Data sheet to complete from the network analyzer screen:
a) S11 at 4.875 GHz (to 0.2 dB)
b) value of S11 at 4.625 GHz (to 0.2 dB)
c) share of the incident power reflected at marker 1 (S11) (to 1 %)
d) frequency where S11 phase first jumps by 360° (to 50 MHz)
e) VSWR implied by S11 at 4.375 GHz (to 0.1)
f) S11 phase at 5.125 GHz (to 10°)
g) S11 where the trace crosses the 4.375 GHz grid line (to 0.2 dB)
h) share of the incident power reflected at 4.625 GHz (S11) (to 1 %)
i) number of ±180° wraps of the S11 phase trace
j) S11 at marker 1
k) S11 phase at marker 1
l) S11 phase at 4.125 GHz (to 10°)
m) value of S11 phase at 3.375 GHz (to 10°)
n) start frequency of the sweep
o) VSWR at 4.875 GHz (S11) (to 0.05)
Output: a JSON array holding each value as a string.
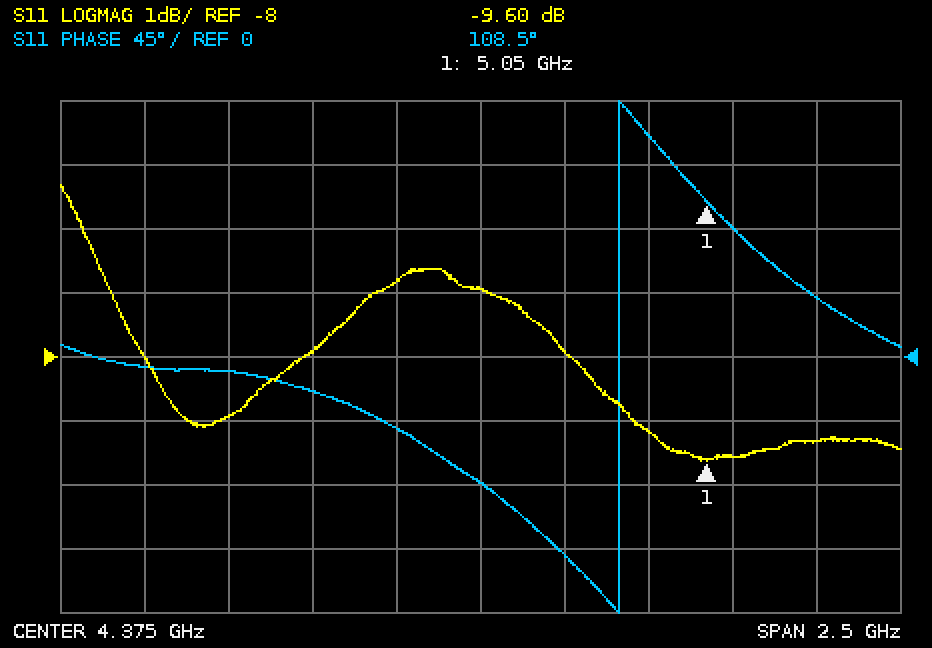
["-9.2 dB", "-8.0 dB", "11 %", "4.80 GHz", "2.6", "90°", "-7.0 dB", "16 %", "1", "-9.60 dB", "108.5°", "-50°", "-10°", "3.125 GHz", "2.05"]
